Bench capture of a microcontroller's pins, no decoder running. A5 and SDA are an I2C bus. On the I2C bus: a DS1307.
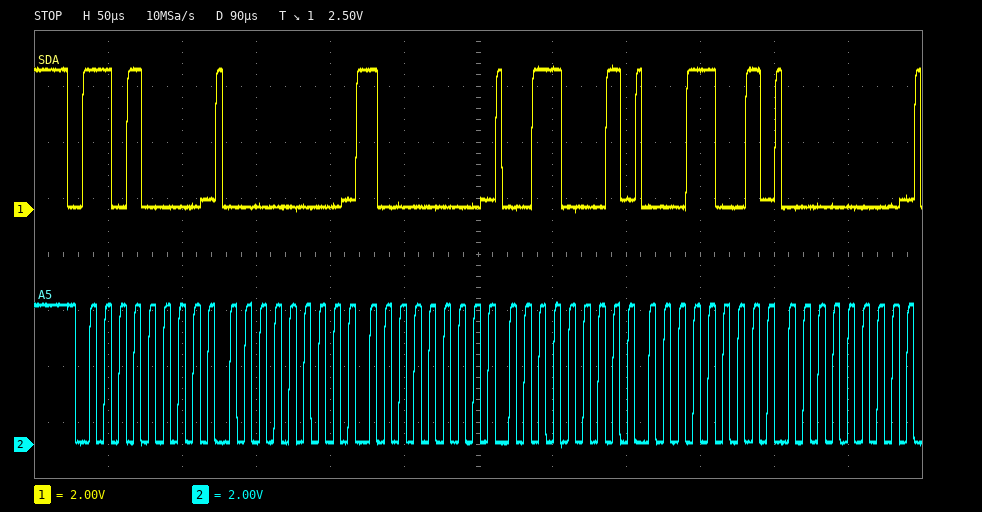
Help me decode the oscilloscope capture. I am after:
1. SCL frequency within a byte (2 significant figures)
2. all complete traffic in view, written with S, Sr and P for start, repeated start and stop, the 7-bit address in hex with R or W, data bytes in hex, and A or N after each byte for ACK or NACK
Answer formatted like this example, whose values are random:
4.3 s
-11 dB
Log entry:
100 kHz
S 68W A 00 A 80 A 31 A 19 A 00 A
